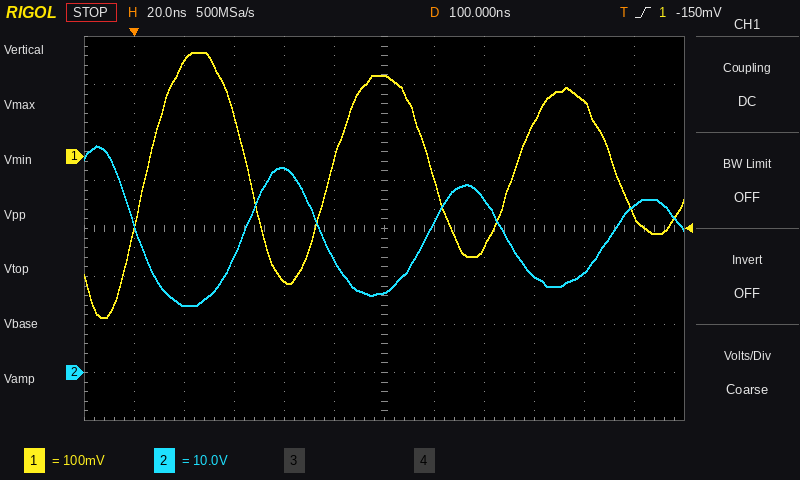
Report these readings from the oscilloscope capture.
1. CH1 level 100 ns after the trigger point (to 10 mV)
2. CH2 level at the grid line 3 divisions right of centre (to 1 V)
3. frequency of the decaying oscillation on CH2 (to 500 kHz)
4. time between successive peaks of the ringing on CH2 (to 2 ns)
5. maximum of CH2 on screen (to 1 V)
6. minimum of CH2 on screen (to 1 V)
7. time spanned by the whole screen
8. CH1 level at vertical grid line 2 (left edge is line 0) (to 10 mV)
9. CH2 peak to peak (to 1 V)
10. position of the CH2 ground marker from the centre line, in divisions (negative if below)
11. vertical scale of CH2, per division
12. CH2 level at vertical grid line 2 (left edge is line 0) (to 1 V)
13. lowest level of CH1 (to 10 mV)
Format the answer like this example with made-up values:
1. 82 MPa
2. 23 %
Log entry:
1. 170 mV
2. 20 V
3. 13.5 MHz
4. 74 ns
5. 47 V
6. 14 V
7. 240 ns
8. 200 mV
9. 33 V
10. -3.0 div
11. 10 V
12. 14 V
13. -340 mV
